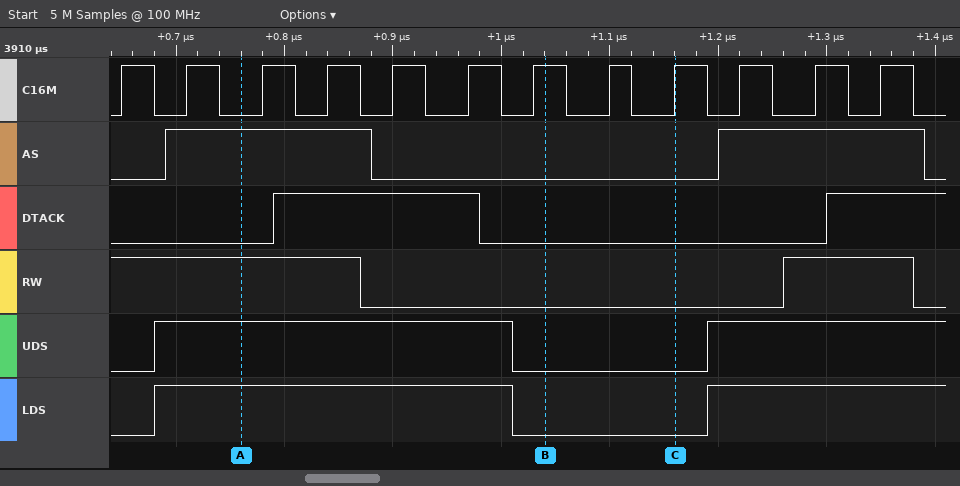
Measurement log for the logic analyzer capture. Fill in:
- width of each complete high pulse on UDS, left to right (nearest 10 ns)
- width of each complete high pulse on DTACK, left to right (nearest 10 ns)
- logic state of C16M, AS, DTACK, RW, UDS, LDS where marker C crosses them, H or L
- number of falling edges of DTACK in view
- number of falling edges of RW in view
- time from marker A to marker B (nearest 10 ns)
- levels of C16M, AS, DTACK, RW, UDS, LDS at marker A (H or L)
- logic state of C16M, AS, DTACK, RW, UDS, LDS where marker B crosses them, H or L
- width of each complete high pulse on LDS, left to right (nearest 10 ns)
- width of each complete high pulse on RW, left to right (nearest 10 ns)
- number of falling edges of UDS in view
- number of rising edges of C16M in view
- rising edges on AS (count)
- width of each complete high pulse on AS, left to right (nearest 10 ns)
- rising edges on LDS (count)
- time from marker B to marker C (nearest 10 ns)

330 ns
190 ns
C16M=H, AS=L, DTACK=L, RW=L, UDS=L, LDS=L
1
2
280 ns
C16M=L, AS=H, DTACK=L, RW=H, UDS=H, LDS=H
C16M=H, AS=L, DTACK=L, RW=L, UDS=L, LDS=L
330 ns
120 ns
1
12
2
190 ns, 190 ns
2
120 ns
